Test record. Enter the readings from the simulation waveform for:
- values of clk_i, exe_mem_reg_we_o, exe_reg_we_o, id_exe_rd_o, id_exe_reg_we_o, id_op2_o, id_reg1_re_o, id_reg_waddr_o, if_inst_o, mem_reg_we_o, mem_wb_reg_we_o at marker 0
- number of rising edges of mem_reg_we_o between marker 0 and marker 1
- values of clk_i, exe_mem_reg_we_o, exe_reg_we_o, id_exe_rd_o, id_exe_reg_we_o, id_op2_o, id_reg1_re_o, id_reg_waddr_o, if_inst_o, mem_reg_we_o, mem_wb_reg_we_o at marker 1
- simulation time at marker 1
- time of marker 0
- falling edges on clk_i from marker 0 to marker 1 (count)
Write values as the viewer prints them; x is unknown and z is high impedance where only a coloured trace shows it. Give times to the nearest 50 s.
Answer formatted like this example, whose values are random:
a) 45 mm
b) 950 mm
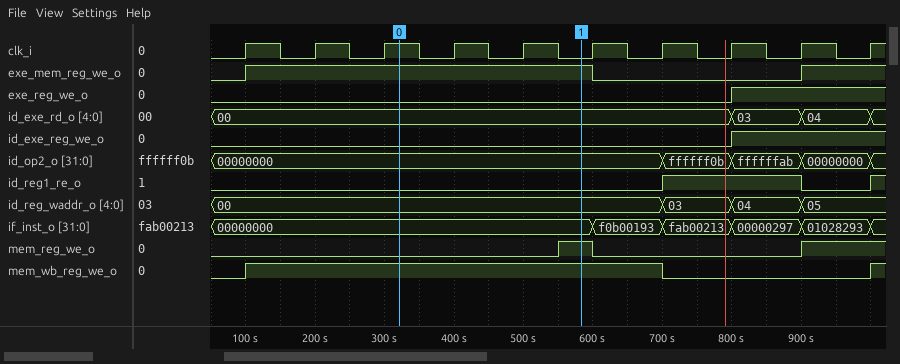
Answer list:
a) clk_i=1, exe_mem_reg_we_o=1, exe_reg_we_o=0, id_exe_rd_o=00, id_exe_reg_we_o=0, id_op2_o=00000000, id_reg1_re_o=0, id_reg_waddr_o=00, if_inst_o=00000000, mem_reg_we_o=0, mem_wb_reg_we_o=1
b) 1
c) clk_i=0, exe_mem_reg_we_o=1, exe_reg_we_o=0, id_exe_rd_o=00, id_exe_reg_we_o=0, id_op2_o=00000000, id_reg1_re_o=0, id_reg_waddr_o=00, if_inst_o=00000000, mem_reg_we_o=1, mem_wb_reg_we_o=1
d) 600 s
e) 300 s
f) 3
